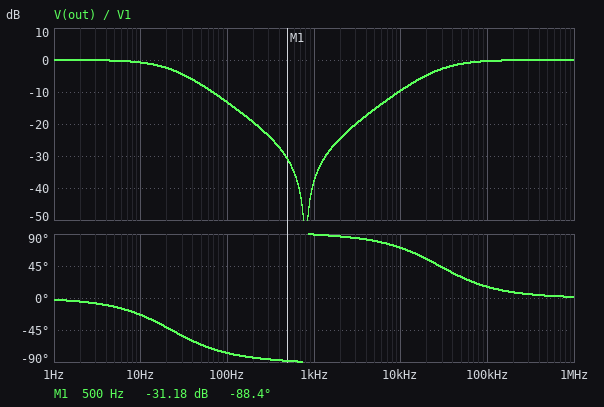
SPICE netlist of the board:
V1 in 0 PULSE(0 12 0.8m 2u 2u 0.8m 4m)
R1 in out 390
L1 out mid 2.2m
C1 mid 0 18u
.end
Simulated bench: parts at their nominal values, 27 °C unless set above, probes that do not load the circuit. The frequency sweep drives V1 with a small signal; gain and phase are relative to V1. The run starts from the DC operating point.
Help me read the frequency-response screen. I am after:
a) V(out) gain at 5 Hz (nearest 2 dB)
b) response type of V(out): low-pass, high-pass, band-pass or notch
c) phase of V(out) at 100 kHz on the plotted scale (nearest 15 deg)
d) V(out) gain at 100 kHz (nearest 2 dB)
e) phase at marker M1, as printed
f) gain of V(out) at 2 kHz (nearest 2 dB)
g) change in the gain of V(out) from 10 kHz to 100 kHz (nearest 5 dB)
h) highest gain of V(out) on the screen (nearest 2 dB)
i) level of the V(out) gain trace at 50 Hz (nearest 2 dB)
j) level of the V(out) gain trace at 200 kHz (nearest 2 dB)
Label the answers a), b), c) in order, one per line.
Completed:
a) 0 dB
b) notch
c) 15 deg
d) 0 dB
e) -88.4 deg
f) -24 dB
g) 10 dB
h) 0 dB
i) -8 dB
j) 0 dB
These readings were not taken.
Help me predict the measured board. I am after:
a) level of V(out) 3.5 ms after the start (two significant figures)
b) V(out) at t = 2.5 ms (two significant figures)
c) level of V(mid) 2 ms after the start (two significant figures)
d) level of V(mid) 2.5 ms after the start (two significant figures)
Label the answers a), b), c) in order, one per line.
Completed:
a) 990 mV
b) 1.1 V
c) 1.2 V
d) 1.1 V
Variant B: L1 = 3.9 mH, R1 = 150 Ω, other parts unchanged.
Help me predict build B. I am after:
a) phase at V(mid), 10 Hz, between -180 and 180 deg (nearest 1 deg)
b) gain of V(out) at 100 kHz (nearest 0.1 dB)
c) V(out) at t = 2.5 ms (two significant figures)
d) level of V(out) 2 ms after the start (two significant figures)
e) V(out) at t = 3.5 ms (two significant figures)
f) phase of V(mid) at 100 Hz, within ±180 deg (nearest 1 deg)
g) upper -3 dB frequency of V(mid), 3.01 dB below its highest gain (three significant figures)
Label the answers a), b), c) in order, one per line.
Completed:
a) -10 deg
b) 0 dB
c) 2.3 V
d) 2.7 V
e) 1.6 V
f) -60 deg
g) 59.5 Hz
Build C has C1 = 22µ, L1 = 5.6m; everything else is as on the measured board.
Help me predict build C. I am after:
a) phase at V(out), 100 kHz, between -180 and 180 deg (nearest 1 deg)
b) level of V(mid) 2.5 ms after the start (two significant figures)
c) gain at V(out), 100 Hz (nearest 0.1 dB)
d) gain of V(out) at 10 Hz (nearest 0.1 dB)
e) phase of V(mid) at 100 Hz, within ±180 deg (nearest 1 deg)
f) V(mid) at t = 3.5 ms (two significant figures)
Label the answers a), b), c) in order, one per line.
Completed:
a) 6 deg
b) 970 mV
c) -15.2 dB
d) -1.1 dB
e) -80 deg
f) 860 mV
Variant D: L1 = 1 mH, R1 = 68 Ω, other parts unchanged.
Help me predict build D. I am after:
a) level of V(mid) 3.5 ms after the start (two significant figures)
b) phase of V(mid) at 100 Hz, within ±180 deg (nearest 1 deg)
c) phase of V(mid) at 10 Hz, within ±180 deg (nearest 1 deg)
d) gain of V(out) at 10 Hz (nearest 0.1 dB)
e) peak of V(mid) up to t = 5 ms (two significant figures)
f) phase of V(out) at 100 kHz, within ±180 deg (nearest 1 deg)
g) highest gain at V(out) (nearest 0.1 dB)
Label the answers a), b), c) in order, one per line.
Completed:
a) 1.2 V
b) -38 deg
c) -4 deg
d) 0 dB
e) 5.8 V
f) 6 deg
g) 0 dB
